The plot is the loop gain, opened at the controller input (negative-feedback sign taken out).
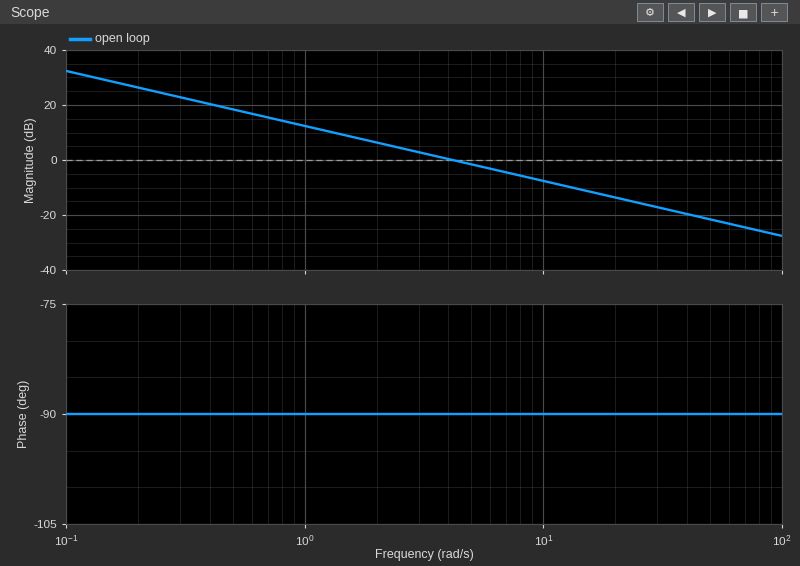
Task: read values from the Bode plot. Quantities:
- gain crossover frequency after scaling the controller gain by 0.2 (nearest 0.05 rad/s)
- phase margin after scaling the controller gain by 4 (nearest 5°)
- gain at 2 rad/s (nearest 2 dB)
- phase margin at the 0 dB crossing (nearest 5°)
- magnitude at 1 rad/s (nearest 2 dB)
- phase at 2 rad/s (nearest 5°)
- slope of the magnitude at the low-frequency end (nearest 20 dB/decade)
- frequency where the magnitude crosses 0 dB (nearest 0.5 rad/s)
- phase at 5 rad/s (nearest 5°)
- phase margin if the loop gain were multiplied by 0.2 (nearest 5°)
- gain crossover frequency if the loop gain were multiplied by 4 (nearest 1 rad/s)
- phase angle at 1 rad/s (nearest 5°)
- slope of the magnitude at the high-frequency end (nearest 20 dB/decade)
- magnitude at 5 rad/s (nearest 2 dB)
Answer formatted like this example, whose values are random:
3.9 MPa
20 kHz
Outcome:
0.85 rad/s
90°
6 dB
90°
12 dB
-90°
-20 dB/decade
4.0 rad/s
-90°
90°
17 rad/s
-90°
-20 dB/decade
-2 dB
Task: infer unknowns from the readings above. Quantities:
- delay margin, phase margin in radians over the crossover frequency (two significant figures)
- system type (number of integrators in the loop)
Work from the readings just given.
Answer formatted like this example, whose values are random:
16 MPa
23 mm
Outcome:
0.39 s
1
